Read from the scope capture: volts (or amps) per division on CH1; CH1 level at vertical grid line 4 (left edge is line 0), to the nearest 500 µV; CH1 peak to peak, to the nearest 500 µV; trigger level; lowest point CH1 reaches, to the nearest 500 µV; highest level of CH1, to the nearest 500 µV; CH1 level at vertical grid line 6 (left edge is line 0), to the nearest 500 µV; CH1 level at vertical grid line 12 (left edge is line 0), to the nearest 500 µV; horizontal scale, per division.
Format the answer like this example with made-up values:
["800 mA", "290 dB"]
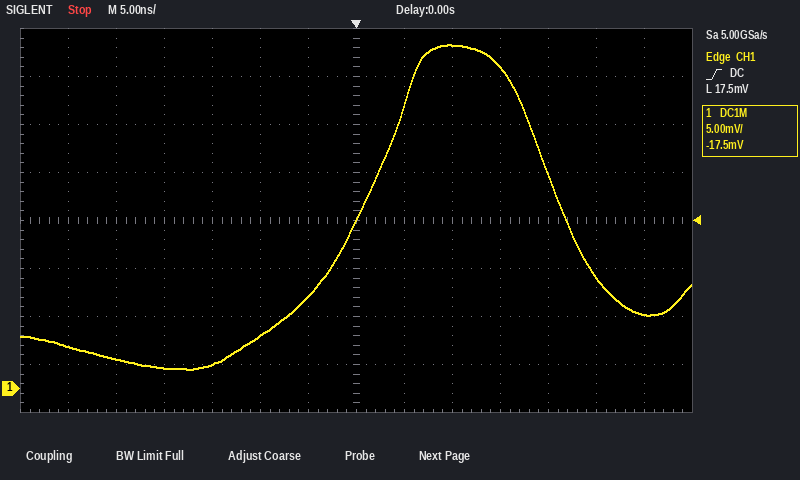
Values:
["5 mV", "2.5 mV", "34.0 mV", "17.5 mV", "2.0 mV", "36.0 mV", "9.5 mV", "11.5 mV", "5 ns"]
